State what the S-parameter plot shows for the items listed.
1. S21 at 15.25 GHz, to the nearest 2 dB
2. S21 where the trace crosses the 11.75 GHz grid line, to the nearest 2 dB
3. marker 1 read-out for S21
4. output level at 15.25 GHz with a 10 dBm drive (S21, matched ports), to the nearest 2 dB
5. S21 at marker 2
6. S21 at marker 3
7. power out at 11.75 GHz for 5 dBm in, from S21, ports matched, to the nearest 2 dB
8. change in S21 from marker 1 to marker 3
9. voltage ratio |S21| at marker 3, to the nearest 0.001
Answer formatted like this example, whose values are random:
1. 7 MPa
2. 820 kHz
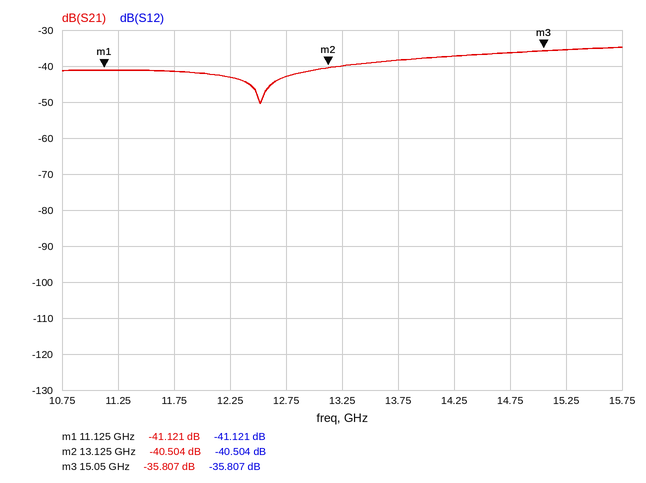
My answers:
1. -36 dB
2. -42 dB
3. -41.121 dB
4. -26 dBm
5. -40.504 dB
6. -35.807 dB
7. -36 dBm
8. 5.314 dB
9. 0.016
